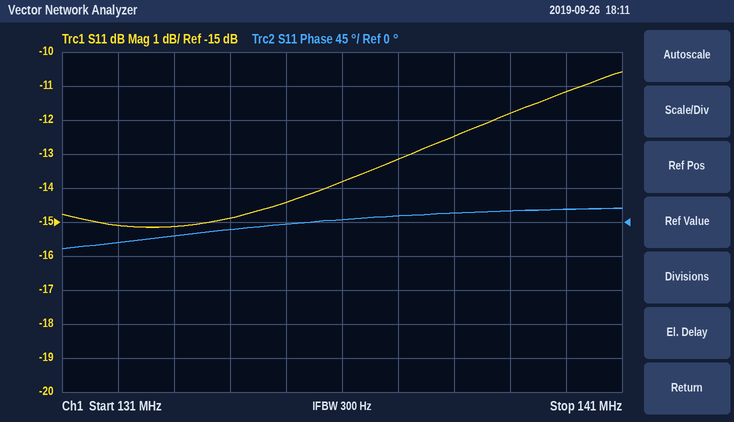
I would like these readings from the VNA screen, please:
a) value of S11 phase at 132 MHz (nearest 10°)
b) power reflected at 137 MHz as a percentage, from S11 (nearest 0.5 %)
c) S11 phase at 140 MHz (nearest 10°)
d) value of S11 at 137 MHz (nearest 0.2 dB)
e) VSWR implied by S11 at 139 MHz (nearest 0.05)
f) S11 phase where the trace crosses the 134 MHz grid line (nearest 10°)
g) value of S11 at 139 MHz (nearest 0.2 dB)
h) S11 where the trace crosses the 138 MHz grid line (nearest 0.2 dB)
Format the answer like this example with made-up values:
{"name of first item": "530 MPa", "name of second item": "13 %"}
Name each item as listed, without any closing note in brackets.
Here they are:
{"value of S11 phase at 132 MHz": "-30°", "power reflected at 137 MHz as a percentage, from S11": "5.0 %", "S11 phase at 140 MHz": "20°", "value of S11 at 137 MHz": "-13.2 dB", "VSWR implied by S11 at 139 MHz": "1.70", "S11 phase where the trace crosses the 134 MHz grid line": "-10°", "value of S11 at 139 MHz": "-11.8 dB", "S11 where the trace crosses the 138 MHz grid line": "-12.4 dB"}
